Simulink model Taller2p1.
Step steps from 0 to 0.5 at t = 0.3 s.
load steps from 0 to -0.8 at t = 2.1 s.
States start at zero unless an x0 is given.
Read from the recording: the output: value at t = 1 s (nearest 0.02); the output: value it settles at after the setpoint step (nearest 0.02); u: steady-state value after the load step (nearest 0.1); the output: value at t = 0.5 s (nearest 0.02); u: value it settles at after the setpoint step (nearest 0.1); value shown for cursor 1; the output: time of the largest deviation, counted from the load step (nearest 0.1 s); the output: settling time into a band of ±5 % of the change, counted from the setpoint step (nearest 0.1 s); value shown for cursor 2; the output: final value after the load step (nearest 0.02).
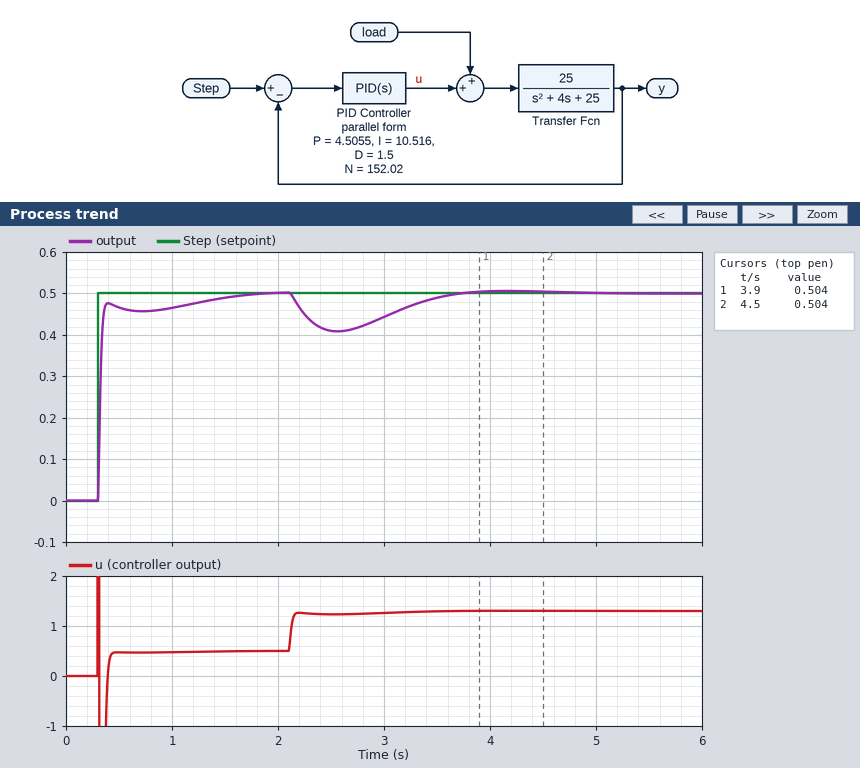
0.46
0.50
1.3
0.46
0.5
0.504
0.5 s
0.9 s
0.504
0.50
